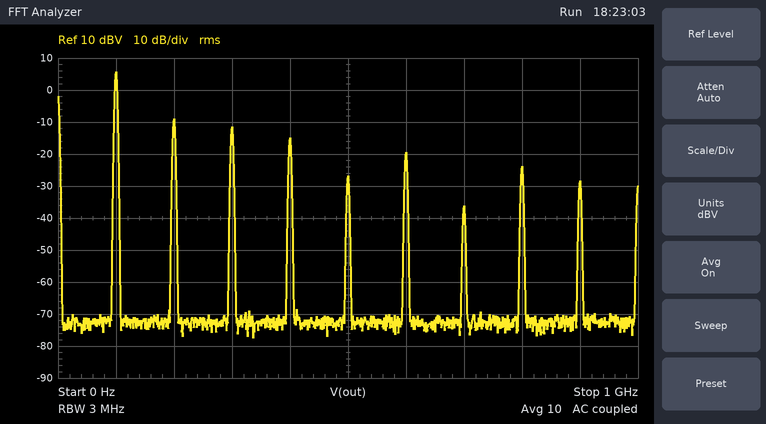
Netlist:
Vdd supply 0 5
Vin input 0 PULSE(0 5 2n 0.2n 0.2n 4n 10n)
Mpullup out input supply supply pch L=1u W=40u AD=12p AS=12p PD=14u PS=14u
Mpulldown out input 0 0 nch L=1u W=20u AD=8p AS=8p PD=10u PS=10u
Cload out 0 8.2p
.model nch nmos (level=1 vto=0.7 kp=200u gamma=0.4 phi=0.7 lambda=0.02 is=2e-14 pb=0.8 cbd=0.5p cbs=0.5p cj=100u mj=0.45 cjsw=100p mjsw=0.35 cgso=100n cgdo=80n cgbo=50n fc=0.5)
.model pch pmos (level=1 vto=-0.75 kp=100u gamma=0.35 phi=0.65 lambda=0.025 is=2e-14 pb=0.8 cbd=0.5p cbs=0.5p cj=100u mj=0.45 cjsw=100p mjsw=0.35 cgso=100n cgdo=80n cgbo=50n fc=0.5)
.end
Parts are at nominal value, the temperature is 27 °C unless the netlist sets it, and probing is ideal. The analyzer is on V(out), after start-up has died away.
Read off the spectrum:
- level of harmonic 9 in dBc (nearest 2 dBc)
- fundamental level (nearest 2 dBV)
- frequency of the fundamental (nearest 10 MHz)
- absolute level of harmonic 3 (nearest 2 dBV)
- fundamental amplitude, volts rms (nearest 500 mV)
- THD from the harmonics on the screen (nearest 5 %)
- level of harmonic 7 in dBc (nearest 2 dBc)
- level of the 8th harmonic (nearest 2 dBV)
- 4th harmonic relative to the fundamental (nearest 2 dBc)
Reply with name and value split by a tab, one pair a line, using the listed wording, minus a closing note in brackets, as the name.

level of harmonic 9 in dBc	-34 dBc
fundamental level	6 dBV
frequency of the fundamental	100 MHz
absolute level of harmonic 3	-12 dBV
fundamental amplitude, volts rms	2.0 V
THD from the harmonics on the screen	25 %
level of harmonic 7 in dBc	-42 dBc
level of the 8th harmonic	-24 dBV
4th harmonic relative to the fundamental	-20 dBc
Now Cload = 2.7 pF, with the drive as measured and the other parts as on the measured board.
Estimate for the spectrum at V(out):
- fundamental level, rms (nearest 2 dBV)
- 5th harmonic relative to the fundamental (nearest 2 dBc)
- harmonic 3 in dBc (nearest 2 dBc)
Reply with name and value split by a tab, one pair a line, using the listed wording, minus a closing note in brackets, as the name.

fundamental level, rms	6 dBV
5th harmonic relative to the fundamental	-30 dBc
harmonic 3 in dBc	-14 dBc
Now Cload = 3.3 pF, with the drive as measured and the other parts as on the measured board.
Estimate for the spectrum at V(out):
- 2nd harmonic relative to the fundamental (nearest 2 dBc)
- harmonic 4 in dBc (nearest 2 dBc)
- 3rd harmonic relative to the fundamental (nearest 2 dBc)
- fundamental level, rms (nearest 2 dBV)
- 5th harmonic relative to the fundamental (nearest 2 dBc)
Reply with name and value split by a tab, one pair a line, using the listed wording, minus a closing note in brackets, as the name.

2nd harmonic relative to the fundamental	-14 dBc
harmonic 4 in dBc	-18 dBc
3rd harmonic relative to the fundamental	-14 dBc
fundamental level, rms	6 dBV
5th harmonic relative to the fundamental	-30 dBc
